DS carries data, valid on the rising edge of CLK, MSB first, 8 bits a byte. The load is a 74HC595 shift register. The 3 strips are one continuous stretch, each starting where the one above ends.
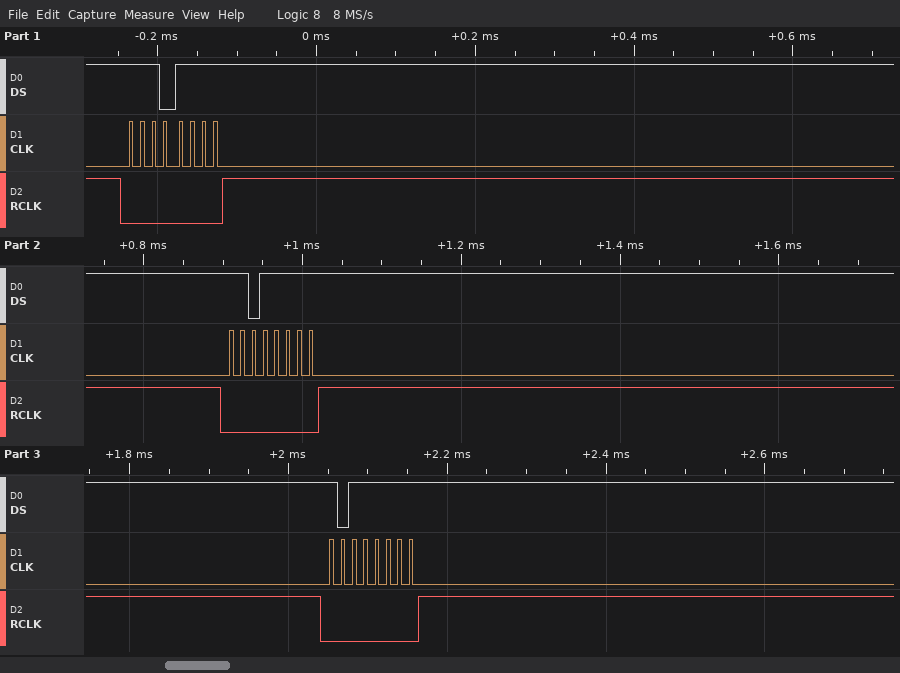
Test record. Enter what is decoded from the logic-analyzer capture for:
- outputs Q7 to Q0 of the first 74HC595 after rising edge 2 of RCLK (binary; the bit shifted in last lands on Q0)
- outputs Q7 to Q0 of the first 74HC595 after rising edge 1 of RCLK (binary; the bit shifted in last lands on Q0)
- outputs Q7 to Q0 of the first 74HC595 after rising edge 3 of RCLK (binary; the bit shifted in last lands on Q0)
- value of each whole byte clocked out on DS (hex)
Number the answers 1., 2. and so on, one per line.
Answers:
1. 11011111
2. 11101111
3. 10111111
4. 0xEF 0xDF 0xBF
